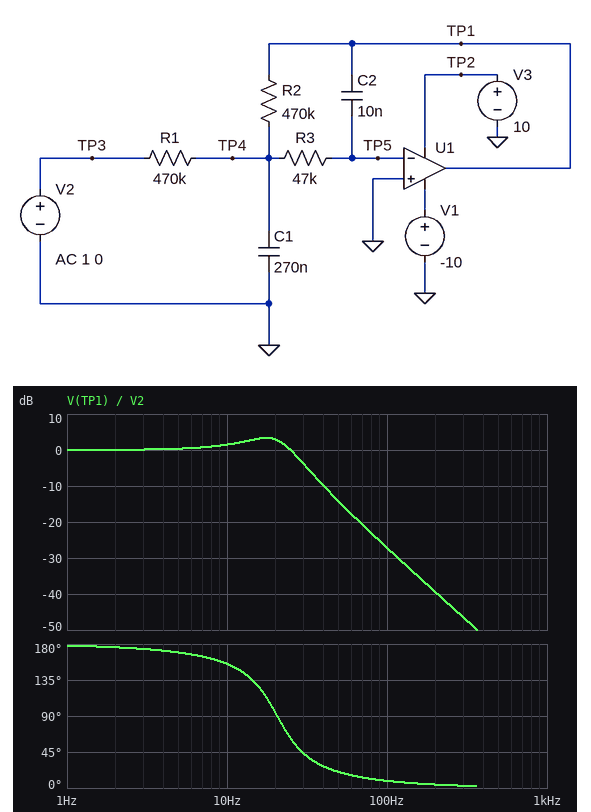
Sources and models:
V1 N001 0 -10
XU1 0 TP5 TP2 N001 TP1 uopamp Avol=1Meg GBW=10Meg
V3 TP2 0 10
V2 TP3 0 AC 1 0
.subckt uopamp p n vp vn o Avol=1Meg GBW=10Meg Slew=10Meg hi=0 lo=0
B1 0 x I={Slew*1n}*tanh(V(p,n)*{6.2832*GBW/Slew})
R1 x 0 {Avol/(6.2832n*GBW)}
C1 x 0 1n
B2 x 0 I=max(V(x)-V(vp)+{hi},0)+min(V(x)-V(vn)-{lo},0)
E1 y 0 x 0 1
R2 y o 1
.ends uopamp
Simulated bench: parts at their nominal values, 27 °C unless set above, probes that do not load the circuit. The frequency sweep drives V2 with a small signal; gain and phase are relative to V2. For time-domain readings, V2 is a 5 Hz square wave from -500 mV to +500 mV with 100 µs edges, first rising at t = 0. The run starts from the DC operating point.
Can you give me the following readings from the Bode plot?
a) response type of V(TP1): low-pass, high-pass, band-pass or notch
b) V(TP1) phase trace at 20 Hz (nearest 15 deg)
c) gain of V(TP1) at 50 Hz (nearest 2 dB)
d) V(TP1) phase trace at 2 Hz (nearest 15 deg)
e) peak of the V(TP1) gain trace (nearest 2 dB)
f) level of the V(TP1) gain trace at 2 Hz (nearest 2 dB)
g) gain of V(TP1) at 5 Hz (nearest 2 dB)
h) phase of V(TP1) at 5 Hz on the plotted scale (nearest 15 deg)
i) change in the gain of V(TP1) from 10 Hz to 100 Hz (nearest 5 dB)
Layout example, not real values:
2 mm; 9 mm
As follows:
low-pass; 90 deg; -14 dB; 180 deg; 4 dB; 0 dB; 0 dB; 165 deg; -30 dB
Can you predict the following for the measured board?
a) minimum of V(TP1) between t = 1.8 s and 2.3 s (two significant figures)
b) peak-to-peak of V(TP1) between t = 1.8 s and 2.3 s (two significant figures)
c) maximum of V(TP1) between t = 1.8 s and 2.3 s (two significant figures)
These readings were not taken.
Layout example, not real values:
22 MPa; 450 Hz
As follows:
-790 mV; 1.6 V; 790 mV
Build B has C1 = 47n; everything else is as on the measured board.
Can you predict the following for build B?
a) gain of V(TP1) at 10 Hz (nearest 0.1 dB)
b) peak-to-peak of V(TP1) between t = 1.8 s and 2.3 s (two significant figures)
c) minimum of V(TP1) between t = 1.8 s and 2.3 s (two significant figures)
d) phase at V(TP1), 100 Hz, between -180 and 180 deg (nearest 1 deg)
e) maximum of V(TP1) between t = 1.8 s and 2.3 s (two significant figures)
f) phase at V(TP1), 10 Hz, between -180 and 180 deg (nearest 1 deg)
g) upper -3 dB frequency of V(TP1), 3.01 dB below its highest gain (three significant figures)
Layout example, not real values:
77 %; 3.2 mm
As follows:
-0.2 dB; 1.0 V; -500 mV; 49 deg; 500 mV; 160 deg; 38.3 Hz
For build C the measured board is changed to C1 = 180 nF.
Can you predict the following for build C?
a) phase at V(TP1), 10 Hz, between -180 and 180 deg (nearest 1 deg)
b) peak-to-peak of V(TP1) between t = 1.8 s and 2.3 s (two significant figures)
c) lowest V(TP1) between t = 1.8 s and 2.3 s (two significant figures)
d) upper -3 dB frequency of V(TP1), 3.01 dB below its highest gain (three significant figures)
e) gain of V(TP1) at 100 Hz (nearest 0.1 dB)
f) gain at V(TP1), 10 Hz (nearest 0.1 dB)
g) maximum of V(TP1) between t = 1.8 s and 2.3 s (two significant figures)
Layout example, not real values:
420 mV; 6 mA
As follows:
157 deg; 1.4 V; -710 mV; 29.9 Hz; -23.6 dB; 0.8 dB; 710 mV
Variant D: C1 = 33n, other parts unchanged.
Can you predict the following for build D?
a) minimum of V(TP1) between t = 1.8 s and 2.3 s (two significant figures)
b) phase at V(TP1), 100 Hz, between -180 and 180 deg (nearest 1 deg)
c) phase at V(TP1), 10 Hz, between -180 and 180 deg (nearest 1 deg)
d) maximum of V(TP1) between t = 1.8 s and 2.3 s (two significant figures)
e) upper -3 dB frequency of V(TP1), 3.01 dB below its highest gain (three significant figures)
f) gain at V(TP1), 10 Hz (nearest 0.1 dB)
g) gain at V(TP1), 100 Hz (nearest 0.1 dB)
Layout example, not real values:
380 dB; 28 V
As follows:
-500 mV; 62 deg; 160 deg; 500 mV; 35.7 Hz; -0.3 dB; -12.1 dB
